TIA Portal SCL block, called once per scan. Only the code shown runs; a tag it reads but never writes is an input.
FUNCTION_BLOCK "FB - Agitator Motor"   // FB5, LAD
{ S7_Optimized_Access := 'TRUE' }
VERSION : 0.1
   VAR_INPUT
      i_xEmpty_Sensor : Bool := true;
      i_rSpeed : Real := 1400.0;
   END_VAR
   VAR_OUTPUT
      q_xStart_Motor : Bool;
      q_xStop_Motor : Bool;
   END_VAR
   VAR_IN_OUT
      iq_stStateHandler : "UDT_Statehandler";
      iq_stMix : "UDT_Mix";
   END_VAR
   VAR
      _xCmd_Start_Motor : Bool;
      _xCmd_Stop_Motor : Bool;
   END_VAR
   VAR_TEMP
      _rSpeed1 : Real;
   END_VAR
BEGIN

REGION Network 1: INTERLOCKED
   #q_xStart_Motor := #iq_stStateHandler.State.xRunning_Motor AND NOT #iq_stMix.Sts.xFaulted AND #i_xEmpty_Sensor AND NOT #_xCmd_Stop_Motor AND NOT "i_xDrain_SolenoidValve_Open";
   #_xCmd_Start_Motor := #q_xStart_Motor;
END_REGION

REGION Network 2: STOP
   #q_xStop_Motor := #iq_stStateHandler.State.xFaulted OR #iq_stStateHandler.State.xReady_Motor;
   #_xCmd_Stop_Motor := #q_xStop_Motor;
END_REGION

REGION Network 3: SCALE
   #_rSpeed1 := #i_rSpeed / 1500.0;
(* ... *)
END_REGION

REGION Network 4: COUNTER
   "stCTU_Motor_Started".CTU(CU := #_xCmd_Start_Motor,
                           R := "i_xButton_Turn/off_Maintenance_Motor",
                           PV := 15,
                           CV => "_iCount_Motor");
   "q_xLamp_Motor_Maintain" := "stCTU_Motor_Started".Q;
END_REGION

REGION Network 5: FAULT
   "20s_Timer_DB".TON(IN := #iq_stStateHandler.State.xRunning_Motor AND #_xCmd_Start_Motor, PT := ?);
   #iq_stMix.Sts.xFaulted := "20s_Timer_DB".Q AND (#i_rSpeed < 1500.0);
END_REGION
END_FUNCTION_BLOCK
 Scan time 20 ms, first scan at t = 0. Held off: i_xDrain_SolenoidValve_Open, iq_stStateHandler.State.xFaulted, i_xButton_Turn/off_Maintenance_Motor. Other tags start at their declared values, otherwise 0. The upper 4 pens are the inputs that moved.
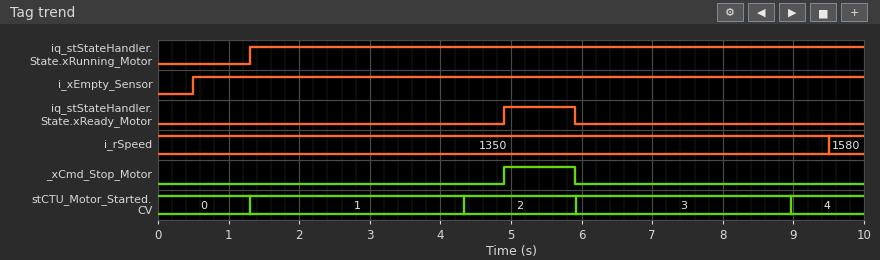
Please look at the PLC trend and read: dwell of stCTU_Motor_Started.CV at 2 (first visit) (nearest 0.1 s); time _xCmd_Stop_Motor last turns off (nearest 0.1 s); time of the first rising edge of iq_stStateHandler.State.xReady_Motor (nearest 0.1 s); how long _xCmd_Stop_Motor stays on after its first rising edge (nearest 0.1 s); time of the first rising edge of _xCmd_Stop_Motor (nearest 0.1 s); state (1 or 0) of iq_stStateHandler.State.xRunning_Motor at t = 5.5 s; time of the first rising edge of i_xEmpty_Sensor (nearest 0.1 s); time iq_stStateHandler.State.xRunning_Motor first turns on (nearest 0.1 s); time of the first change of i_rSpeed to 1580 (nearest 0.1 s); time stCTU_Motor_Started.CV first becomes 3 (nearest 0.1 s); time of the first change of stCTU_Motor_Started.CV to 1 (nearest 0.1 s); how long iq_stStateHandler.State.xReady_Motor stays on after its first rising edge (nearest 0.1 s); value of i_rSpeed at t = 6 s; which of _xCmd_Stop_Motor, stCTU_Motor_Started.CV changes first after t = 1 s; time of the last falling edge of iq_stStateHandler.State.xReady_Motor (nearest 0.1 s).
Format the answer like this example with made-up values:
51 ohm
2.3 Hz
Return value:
1.6 s
5.9 s
4.9 s
1.0 s
4.9 s
1
0.5 s
1.3 s
9.5 s
5.9 s
1.3 s
1.0 s
1350
stCTU_Motor_Started.CV
5.9 s
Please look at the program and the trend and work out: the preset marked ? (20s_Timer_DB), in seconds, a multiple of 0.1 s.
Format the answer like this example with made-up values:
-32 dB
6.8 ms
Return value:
3.0 s
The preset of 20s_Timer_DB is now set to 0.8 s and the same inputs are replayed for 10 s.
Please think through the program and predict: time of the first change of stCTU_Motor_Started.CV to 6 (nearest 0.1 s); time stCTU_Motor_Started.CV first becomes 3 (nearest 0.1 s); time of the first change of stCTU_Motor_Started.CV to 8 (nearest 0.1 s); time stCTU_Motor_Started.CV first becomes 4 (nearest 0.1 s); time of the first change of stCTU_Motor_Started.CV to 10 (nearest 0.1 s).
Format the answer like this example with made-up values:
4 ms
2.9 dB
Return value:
5.9 s
3.0 s
7.6 s
3.8 s
9.3 s
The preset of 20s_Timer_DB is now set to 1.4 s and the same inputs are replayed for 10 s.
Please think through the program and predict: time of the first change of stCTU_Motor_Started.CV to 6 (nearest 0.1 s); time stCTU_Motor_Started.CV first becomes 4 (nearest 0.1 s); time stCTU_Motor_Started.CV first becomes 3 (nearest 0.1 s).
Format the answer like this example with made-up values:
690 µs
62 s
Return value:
8.8 s
5.9 s
4.2 s
